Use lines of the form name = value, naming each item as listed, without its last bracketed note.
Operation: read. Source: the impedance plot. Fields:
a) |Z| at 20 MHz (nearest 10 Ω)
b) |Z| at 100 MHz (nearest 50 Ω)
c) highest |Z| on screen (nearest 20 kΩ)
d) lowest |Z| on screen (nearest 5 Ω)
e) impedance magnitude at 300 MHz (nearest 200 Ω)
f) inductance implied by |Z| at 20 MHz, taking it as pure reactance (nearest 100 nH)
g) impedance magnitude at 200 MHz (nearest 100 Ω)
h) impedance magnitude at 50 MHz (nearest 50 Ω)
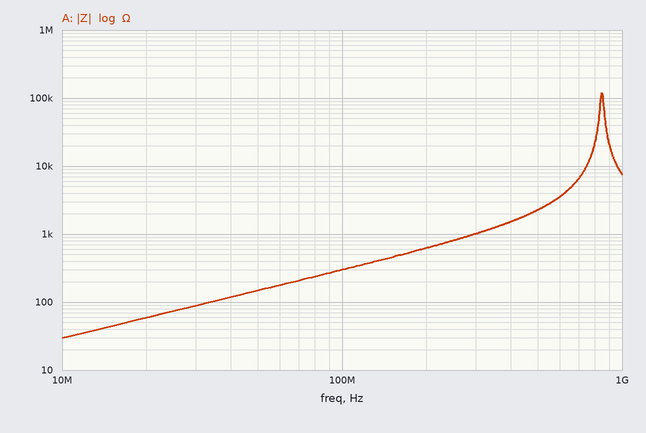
|Z| at 20 MHz = 60 Ω
|Z| at 100 MHz = 300 Ω
highest |Z| on screen = 120 kΩ
lowest |Z| on screen = 30 Ω
impedance magnitude at 300 MHz = 1.0 kΩ
inductance implied by |Z| at 20 MHz, taking it as pure reactance = 500 nH
impedance magnitude at 200 MHz = 600 Ω
impedance magnitude at 50 MHz = 150 Ω
